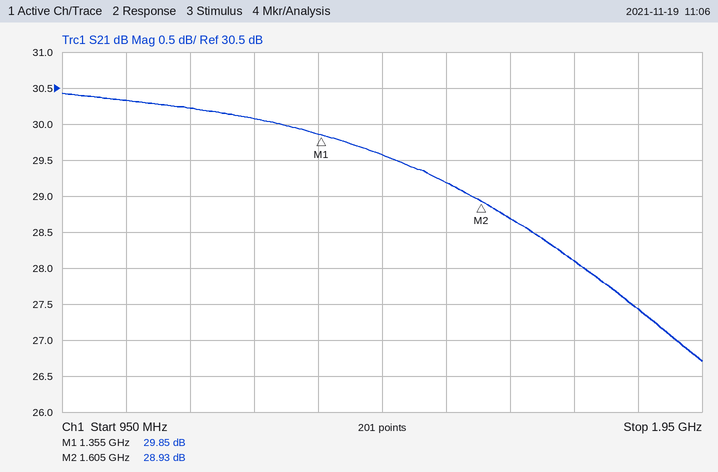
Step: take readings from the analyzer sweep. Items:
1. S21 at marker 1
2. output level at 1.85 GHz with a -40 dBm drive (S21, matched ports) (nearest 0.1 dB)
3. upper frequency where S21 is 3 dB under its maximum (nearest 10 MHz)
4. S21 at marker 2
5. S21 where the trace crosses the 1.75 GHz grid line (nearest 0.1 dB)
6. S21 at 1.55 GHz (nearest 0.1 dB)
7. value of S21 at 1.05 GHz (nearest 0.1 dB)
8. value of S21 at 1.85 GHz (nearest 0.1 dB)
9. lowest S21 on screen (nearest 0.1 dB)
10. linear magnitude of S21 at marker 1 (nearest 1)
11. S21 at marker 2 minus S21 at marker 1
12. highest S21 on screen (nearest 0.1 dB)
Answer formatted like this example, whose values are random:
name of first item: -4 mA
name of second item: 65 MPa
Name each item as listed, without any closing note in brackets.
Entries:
S21 at marker 1: 29.85 dB
output level at 1.85 GHz with a -40 dBm drive (S21, matched ports): -12.6 dBm
upper frequency where S21 is 3 dB under its maximum: 1.85 GHz
S21 at marker 2: 28.93 dB
S21 where the trace crosses the 1.75 GHz grid line: 28.1 dB
S21 at 1.55 GHz: 29.2 dB
value of S21 at 1.05 GHz: 30.3 dB
value of S21 at 1.85 GHz: 27.4 dB
lowest S21 on screen: 26.7 dB
linear magnitude of S21 at marker 1: 31
S21 at marker 2 minus S21 at marker 1: -0.92 dB
highest S21 on screen: 30.4 dB
